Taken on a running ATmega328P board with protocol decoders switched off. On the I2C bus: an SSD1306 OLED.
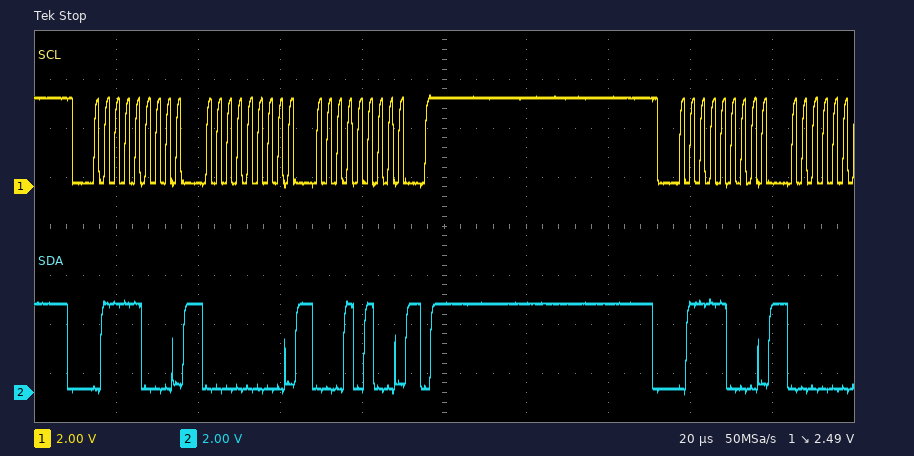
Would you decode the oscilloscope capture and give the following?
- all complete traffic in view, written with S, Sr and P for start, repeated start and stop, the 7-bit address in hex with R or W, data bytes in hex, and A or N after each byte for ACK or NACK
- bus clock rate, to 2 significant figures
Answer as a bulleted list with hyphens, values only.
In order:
- S 3CW A 00 A 14 A P S 3CW A
- 400 kHz
